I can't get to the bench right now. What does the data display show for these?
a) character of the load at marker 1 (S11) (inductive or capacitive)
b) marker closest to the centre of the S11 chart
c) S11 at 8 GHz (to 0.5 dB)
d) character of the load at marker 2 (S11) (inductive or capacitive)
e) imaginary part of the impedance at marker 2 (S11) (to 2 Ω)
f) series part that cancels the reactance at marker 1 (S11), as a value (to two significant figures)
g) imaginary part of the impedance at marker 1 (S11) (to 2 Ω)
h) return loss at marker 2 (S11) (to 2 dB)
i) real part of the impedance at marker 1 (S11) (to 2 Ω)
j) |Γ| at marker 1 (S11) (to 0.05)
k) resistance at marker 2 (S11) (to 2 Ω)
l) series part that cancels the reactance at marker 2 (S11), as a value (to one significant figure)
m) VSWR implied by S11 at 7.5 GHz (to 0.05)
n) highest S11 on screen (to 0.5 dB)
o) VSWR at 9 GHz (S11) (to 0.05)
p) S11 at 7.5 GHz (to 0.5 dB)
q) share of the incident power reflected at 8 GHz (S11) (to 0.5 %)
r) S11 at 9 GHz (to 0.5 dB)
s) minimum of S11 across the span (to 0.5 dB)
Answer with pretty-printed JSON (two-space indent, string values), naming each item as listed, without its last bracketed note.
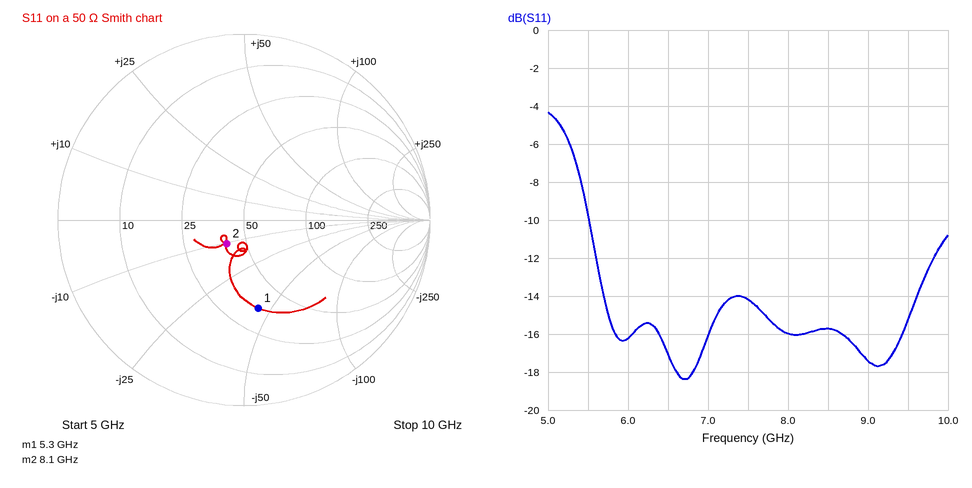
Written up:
{
  "character of the load at marker 1 (S11)": "capacitive",
  "marker closest to the centre of the S11 chart": "marker 2",
  "S11 at 8 GHz": "-16.0 dB",
  "character of the load at marker 2 (S11)": "capacitive",
  "imaginary part of the impedance at marker 2 (S11)": "-10 Ω",
  "series part that cancels the reactance at marker 1 (S11), as a value": "1.3 nH",
  "imaginary part of the impedance at marker 1 (S11)": "-44 Ω",
  "return loss at marker 2 (S11)": "16 dB",
  "real part of the impedance at marker 1 (S11)": "36 Ω",
  "|Γ| at marker 1 (S11)": "0.50",
  "resistance at marker 2 (S11)": "40 Ω",
  "series part that cancels the reactance at marker 2 (S11), as a value": "200 pH",
  "VSWR implied by S11 at 7.5 GHz": "1.50",
  "highest S11 on screen": "-4.5 dB",
  "VSWR at 9 GHz (S11)": "1.30",
  "S11 at 7.5 GHz": "-14.0 dB",
  "share of the incident power reflected at 8 GHz (S11)": "2.5 %",
  "S11 at 9 GHz": "-17.5 dB",
  "minimum of S11 across the span": "-18.5 dB"
}
